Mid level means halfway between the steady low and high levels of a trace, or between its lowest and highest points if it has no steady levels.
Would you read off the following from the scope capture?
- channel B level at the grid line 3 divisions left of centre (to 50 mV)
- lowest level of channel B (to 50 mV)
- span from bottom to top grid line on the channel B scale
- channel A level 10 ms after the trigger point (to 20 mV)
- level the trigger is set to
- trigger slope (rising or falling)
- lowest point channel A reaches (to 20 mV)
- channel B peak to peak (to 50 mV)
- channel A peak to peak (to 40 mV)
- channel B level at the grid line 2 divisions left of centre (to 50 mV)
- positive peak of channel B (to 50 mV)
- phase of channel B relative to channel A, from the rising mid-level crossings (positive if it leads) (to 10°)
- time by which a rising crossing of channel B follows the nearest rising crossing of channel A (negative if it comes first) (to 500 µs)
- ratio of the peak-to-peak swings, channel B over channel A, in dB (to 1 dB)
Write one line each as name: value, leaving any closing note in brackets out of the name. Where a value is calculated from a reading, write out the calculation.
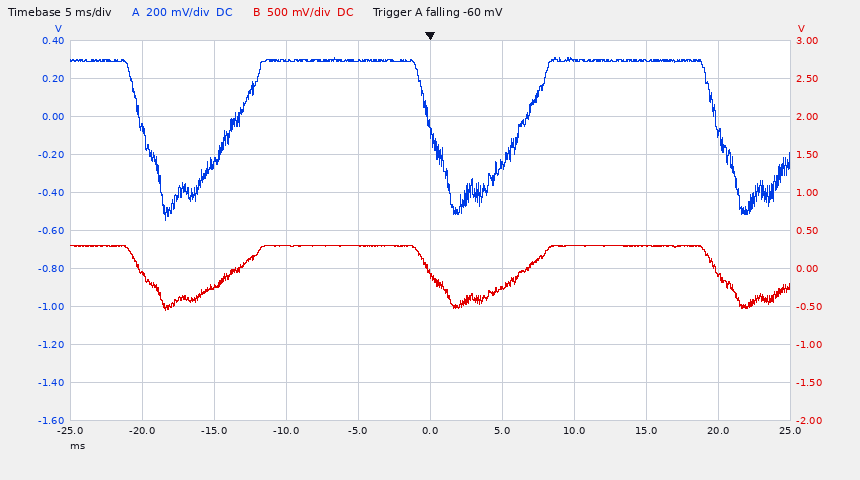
channel B level at the grid line 3 divisions left of centre: -250 mV
lowest level of channel B: -550 mV
span from bottom to top grid line on the channel B scale: 5 V
channel A level 10 ms after the trigger point: 300 mV
level the trigger is set to: -60 mV
trigger slope: falling
lowest point channel A reaches: -540 mV
channel B peak to peak: 300 mV − (-550 mV) = 850 mV
channel A peak to peak: 840 mV
channel B level at the grid line 2 divisions left of centre: 300 mV
positive peak of channel B: 300 mV
phase of channel B relative to channel A, from the rising mid-level crossings (positive if it leads): 0°
time by which a rising crossing of channel B follows the nearest rising crossing of channel A (negative if it comes first): 0.0 ms
ratio of the peak-to-peak swings, channel B over channel A, in dB: 20 log10(850 mV / 840 mV) ≈ 0 dB
